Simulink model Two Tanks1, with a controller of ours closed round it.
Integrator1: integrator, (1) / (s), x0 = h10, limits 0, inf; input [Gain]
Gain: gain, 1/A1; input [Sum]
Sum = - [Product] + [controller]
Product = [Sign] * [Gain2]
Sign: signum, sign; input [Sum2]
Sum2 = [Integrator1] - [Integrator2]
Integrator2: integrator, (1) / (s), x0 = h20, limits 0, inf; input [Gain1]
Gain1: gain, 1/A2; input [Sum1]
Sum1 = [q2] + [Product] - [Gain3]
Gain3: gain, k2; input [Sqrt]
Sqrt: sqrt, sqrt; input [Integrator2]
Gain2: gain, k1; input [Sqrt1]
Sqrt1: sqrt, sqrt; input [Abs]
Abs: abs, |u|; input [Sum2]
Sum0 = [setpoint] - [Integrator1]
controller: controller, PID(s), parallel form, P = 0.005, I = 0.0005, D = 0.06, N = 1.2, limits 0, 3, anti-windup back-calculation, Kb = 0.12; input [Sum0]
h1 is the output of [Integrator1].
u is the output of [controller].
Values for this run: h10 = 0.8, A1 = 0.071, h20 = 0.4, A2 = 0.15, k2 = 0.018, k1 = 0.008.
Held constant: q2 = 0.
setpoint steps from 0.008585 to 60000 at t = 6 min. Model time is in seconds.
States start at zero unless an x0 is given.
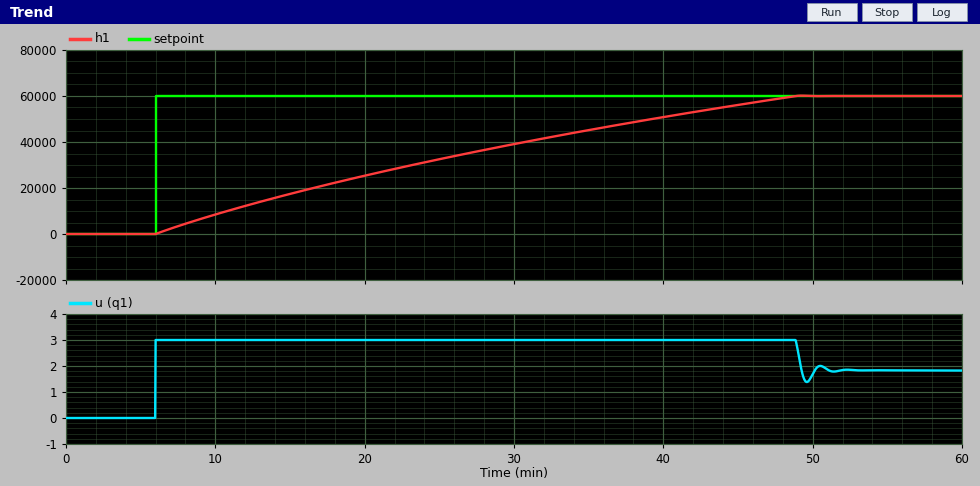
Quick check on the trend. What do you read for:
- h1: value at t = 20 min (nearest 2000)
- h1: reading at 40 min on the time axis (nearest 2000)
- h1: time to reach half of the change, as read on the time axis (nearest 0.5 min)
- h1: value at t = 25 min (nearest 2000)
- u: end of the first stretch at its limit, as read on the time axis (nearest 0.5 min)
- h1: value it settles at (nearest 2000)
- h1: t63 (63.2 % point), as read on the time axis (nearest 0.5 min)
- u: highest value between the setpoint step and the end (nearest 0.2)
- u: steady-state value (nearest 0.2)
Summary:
26000
50000
23.0 min
32000
49.0 min
60000
29.0 min
3.0
1.8
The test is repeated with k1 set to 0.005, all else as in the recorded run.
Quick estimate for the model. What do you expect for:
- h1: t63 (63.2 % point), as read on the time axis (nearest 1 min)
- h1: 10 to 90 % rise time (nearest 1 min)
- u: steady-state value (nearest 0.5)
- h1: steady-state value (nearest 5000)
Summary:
25 min
26 min
1.0
60000
